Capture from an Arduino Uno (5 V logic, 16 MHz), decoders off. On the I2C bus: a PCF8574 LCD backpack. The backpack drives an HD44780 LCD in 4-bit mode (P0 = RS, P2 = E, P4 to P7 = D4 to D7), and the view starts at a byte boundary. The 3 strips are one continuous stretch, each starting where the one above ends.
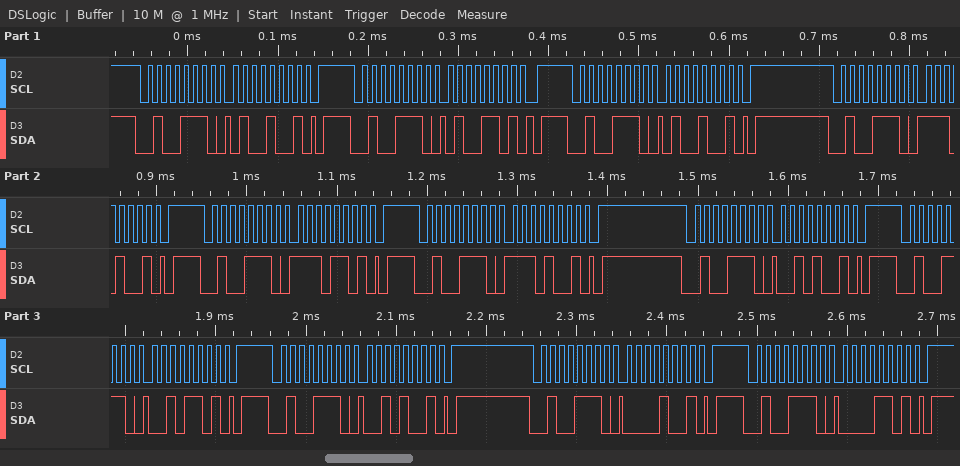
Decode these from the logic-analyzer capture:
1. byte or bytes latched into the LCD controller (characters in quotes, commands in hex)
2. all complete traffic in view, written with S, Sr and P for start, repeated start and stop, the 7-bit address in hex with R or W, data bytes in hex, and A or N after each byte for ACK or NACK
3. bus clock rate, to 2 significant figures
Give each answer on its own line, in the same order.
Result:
'N'
S 27W A 49 A P S 27W A 4D A P S 27W A 49 A P S 27W A E9 A P S 27W A ED A P S 27W A E9 A P S 27W A 29 A P S 27W A 2D A P S 27W A 29 A P S 27W A 09 A P S 27W A 0D A P
100 kHz
